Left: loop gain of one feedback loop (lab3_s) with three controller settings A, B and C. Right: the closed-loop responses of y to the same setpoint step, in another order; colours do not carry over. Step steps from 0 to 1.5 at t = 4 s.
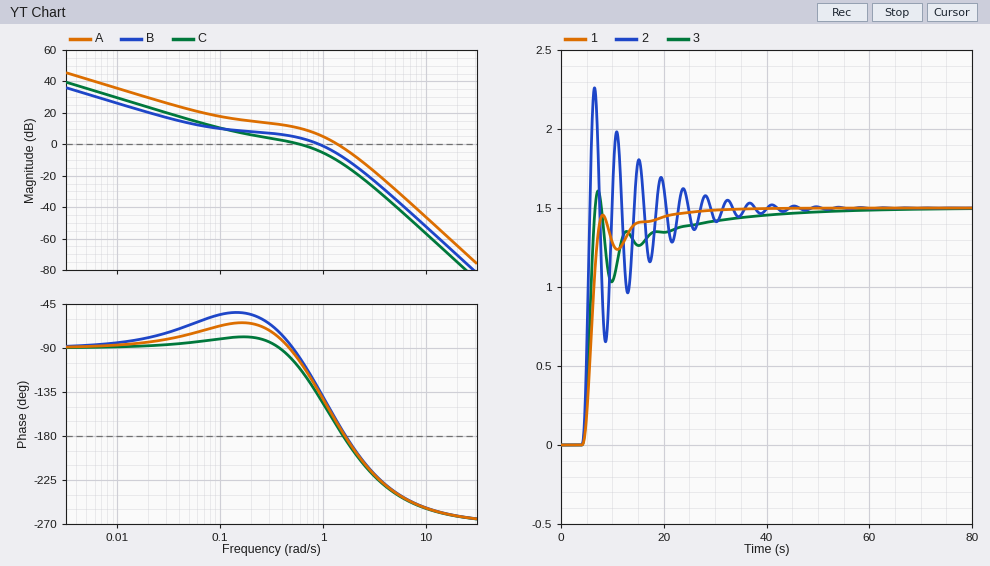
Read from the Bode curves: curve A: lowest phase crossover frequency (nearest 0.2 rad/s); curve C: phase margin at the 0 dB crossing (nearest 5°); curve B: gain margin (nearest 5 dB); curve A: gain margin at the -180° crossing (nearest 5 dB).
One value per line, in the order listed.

1.6 rad/s
70°
10 dB
5 dB
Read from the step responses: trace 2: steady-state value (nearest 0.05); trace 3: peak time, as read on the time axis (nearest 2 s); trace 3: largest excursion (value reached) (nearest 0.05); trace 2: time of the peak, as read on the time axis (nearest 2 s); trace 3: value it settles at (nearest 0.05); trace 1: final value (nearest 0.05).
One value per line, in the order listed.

1.50
8 s
1.60
6 s
1.50
1.50
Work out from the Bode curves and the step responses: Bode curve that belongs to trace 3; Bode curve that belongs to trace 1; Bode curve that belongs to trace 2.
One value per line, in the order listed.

B
C
A
